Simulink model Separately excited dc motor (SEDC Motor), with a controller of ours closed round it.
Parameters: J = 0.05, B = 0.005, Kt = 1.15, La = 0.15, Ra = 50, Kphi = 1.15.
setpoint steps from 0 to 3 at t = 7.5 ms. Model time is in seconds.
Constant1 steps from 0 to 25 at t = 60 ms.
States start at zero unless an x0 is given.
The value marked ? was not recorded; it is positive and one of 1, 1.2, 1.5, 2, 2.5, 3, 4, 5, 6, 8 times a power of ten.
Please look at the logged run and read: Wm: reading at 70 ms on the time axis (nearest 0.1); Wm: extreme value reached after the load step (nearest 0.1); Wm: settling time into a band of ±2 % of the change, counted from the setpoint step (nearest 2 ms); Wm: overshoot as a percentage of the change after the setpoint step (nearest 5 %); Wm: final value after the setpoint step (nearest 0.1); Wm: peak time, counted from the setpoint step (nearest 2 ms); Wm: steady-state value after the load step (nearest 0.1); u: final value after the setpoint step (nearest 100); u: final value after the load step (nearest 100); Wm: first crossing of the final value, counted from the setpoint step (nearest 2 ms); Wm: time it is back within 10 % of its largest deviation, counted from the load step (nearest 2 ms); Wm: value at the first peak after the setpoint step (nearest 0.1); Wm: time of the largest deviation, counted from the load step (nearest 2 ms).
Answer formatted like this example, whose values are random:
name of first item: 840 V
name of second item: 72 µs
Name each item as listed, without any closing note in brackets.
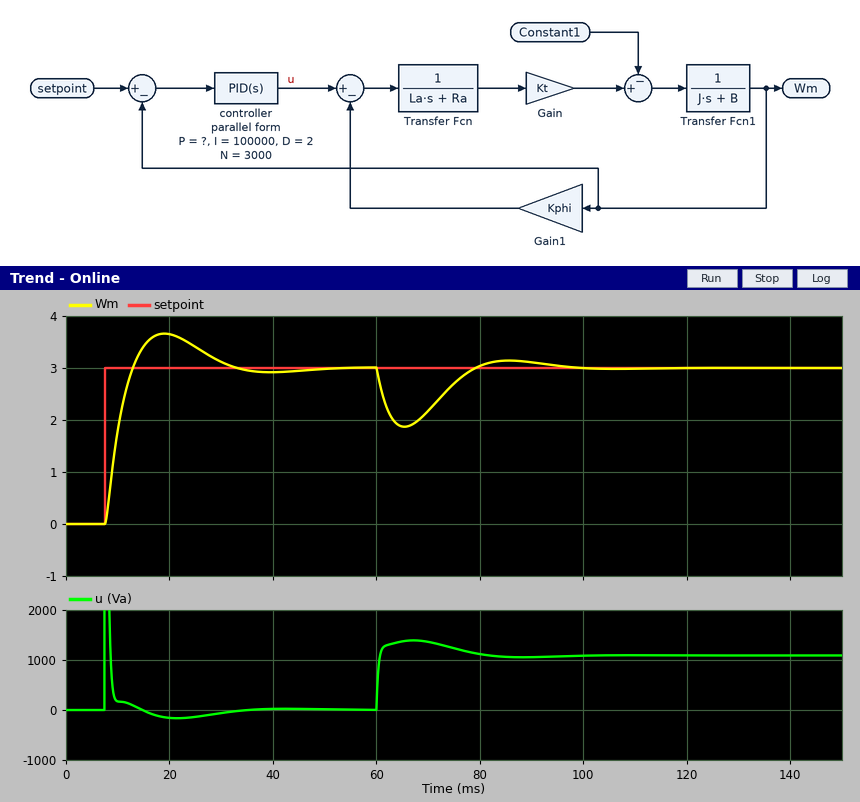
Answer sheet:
Wm: reading at 70 ms on the time axis: 2.2
Wm: extreme value reached after the load step: 1.9
Wm: settling time into a band of ±2 % of the change, counted from the setpoint step: 36 ms
Wm: overshoot as a percentage of the change after the setpoint step: 20 %
Wm: final value after the setpoint step: 3.0
Wm: peak time, counted from the setpoint step: 12 ms
Wm: steady-state value after the load step: 3.0
u: final value after the setpoint step: 0
u: final value after the load step: 1100
Wm: first crossing of the final value, counted from the setpoint step: 6 ms
Wm: time it is back within 10 % of its largest deviation, counted from the load step: 30 ms
Wm: value at the first peak after the setpoint step: 3.7
Wm: time of the largest deviation, counted from the load step: 6 ms
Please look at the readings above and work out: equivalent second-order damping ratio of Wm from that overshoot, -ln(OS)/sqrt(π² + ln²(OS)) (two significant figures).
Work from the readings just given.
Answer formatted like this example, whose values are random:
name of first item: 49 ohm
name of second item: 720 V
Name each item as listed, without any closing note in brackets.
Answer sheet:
equivalent second-order damping ratio of Wm from that overshoot, -ln(OS)/sqrt(π² + ln²(OS)): 0.46
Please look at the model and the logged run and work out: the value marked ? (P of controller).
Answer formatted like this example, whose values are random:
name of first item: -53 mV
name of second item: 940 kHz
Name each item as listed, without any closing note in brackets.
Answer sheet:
the value marked ?: 800
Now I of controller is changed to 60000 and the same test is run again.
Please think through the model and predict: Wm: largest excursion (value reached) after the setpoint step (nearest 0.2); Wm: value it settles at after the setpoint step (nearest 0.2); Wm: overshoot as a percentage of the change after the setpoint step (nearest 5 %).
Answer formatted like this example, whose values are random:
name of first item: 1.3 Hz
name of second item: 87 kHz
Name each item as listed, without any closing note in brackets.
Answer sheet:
Wm: largest excursion (value reached) after the setpoint step: 3.4
Wm: value it settles at after the setpoint step: 3.0
Wm: overshoot as a percentage of the change after the setpoint step: 15 %
